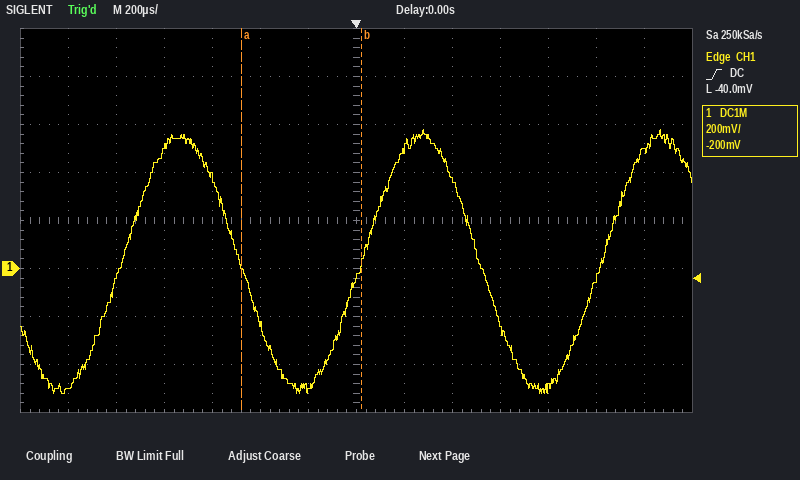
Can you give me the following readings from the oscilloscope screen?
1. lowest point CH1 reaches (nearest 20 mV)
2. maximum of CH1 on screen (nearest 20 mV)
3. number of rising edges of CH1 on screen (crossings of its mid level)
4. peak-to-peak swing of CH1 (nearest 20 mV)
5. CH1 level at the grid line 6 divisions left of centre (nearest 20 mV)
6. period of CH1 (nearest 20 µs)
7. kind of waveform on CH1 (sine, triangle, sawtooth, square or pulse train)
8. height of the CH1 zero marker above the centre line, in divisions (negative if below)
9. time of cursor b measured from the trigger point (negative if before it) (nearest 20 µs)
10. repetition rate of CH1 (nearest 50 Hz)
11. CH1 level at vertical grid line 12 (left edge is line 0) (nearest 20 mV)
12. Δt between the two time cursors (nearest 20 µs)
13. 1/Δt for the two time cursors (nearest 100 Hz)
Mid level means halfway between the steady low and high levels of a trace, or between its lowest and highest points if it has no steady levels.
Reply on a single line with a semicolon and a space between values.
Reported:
-520 mV; 580 mV; 3; 1.10 V; -500 mV; 1.00 ms; sine; -1.0 div; +20 µs; 1.00 kHz; -40 mV; 500 µs; 2.0 kHz
